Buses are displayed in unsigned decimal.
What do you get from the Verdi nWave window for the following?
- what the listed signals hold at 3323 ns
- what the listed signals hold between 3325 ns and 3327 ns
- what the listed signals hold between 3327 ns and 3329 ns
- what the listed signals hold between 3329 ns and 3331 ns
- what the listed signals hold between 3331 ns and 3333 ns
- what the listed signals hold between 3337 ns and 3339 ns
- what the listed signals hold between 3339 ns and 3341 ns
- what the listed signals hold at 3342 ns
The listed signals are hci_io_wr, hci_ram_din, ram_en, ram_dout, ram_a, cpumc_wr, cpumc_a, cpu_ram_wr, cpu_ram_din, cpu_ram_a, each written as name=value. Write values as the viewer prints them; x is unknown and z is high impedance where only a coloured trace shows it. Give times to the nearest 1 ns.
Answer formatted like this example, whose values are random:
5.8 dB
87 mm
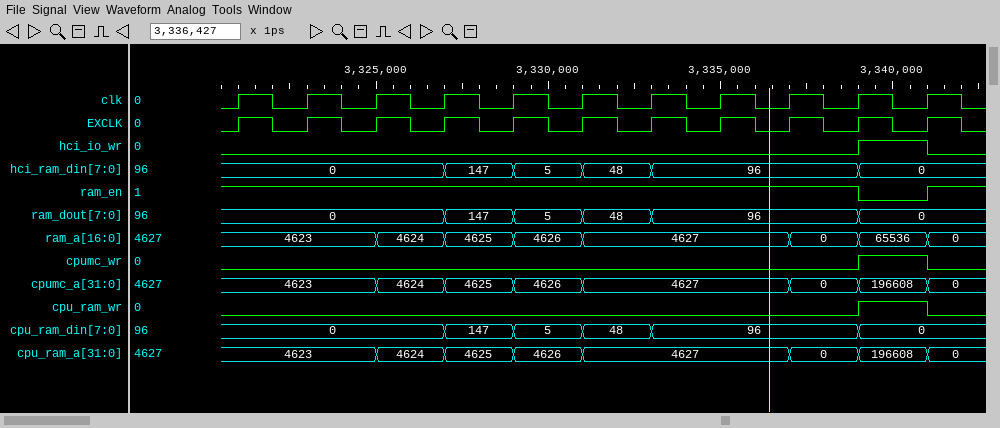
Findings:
hci_io_wr=0, hci_ram_din=0, ram_en=1, ram_dout=0, ram_a=4623, cpumc_wr=0, cpumc_a=4623, cpu_ram_wr=0, cpu_ram_din=0, cpu_ram_a=4623
hci_io_wr=0, hci_ram_din=0, ram_en=1, ram_dout=0, ram_a=4624, cpumc_wr=0, cpumc_a=4624, cpu_ram_wr=0, cpu_ram_din=0, cpu_ram_a=4624
hci_io_wr=0, hci_ram_din=147, ram_en=1, ram_dout=147, ram_a=4625, cpumc_wr=0, cpumc_a=4625, cpu_ram_wr=0, cpu_ram_din=147, cpu_ram_a=4625
hci_io_wr=0, hci_ram_din=5, ram_en=1, ram_dout=5, ram_a=4626, cpumc_wr=0, cpumc_a=4626, cpu_ram_wr=0, cpu_ram_din=5, cpu_ram_a=4626
hci_io_wr=0, hci_ram_din=48, ram_en=1, ram_dout=48, ram_a=4627, cpumc_wr=0, cpumc_a=4627, cpu_ram_wr=0, cpu_ram_din=48, cpu_ram_a=4627
hci_io_wr=0, hci_ram_din=96, ram_en=1, ram_dout=96, ram_a=0, cpumc_wr=0, cpumc_a=0, cpu_ram_wr=0, cpu_ram_din=96, cpu_ram_a=0
hci_io_wr=1, hci_ram_din=0, ram_en=0, ram_dout=0, ram_a=65536, cpumc_wr=1, cpumc_a=196608, cpu_ram_wr=1, cpu_ram_din=0, cpu_ram_a=196608
hci_io_wr=0, hci_ram_din=0, ram_en=1, ram_dout=0, ram_a=0, cpumc_wr=0, cpumc_a=0, cpu_ram_wr=0, cpu_ram_din=0, cpu_ram_a=0
